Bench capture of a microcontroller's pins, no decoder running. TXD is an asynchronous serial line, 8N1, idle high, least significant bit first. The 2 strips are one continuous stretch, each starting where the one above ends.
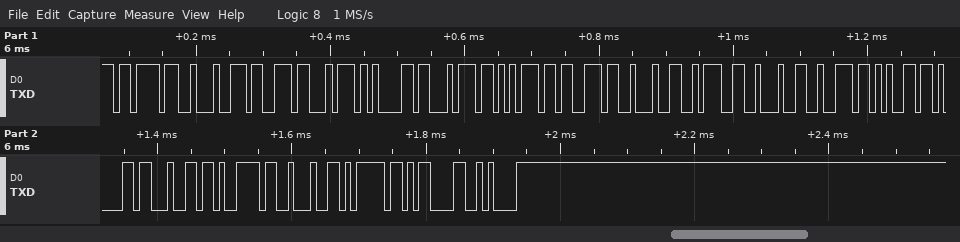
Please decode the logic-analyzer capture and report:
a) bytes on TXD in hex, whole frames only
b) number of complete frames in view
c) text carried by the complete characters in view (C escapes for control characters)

7B 22 73 74 61 74 75 73 22 3A 22 72 65 61 64 79 22 7D 0D 0A
20
"{\"status\":\"ready\"}\r\n"
